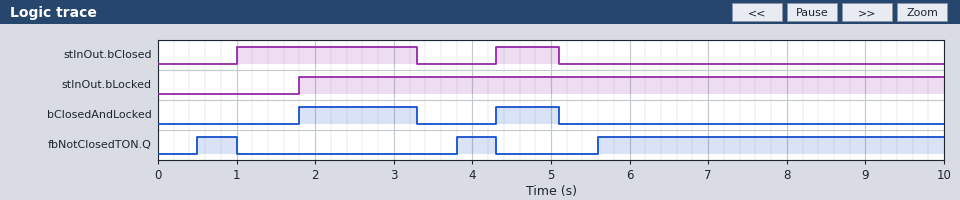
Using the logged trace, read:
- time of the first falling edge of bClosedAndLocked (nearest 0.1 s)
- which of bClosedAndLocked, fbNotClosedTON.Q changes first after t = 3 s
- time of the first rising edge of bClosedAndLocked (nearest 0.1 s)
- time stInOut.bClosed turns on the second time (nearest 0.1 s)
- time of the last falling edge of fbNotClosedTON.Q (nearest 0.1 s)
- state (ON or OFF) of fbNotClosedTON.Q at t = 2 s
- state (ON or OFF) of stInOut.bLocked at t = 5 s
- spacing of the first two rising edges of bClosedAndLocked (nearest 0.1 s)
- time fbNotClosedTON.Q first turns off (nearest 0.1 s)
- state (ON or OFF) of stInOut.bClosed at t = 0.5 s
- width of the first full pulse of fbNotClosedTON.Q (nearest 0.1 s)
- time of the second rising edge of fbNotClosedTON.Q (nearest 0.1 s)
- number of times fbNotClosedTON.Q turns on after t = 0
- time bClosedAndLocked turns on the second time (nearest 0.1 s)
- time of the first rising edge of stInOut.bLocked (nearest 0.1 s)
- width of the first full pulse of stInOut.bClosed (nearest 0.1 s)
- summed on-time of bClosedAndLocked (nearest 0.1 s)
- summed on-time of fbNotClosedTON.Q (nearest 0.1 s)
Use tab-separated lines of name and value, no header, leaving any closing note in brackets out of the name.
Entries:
time of the first falling edge of bClosedAndLocked	3.3 s
which of bClosedAndLocked, fbNotClosedTON.Q changes first after t = 3 s	bClosedAndLocked
time of the first rising edge of bClosedAndLocked	1.8 s
time stInOut.bClosed turns on the second time	4.3 s
time of the last falling edge of fbNotClosedTON.Q	4.3 s
state (ON or OFF) of fbNotClosedTON.Q at t = 2 s	OFF
state (ON or OFF) of stInOut.bLocked at t = 5 s	ON
spacing of the first two rising edges of bClosedAndLocked	2.5 s
time fbNotClosedTON.Q first turns off	1.0 s
state (ON or OFF) of stInOut.bClosed at t = 0.5 s	OFF
width of the first full pulse of fbNotClosedTON.Q	0.5 s
time of the second rising edge of fbNotClosedTON.Q	3.8 s
number of times fbNotClosedTON.Q turns on after t = 0	3
time bClosedAndLocked turns on the second time	4.3 s
time of the first rising edge of stInOut.bLocked	1.8 s
width of the first full pulse of stInOut.bClosed	2.3 s
summed on-time of bClosedAndLocked	2.3 s
summed on-time of fbNotClosedTON.Q	5.4 s
